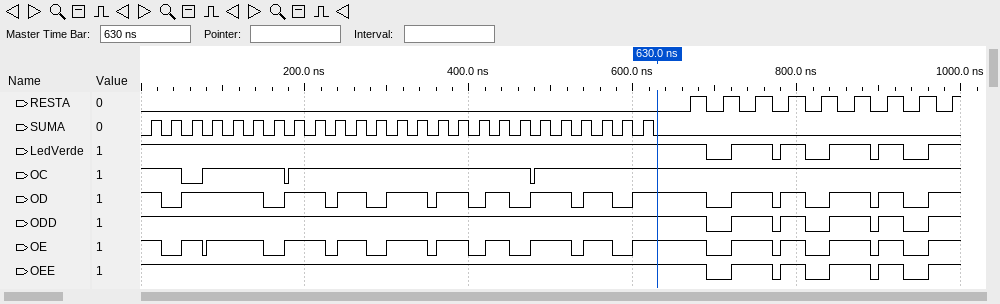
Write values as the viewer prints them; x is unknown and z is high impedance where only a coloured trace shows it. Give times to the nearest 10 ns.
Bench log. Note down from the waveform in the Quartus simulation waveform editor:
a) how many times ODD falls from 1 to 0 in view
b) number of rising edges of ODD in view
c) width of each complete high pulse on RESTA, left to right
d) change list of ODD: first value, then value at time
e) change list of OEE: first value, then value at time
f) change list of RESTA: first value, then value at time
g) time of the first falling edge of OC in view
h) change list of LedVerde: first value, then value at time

5
5
20 ns, 20 ns, 20 ns, 20 ns, 20 ns, 20 ns, 20 ns, 20 ns
1, 0 at 690 ns, 1 at 720 ns, 0 at 770 ns, 1 at 780 ns, 0 at 810 ns, 1 at 840 ns, 0 at 890 ns, 1 at 900 ns, 0 at 930 ns, 1 at 960 ns
1, 0 at 690 ns, 1 at 720 ns, 0 at 770 ns, 1 at 780 ns, 0 at 810 ns, 1 at 840 ns, 0 at 890 ns, 1 at 900 ns, 0 at 930 ns, 1 at 960 ns
0, 1 at 670 ns, 0 at 690 ns, 1 at 710 ns, 0 at 730 ns, 1 at 750 ns, 0 at 770 ns, 1 at 790 ns, 0 at 810 ns, 1 at 830 ns, 0 at 850 ns, 1 at 870 ns, 0 at 890 ns, 1 at 910 ns, 0 at 930 ns, 1 at 950 ns, 0 at 970 ns, 1 at 990 ns
50 ns
1, 0 at 690 ns, 1 at 720 ns, 0 at 770 ns, 1 at 780 ns, 0 at 810 ns, 1 at 840 ns, 0 at 890 ns, 1 at 900 ns, 0 at 930 ns, 1 at 960 ns
